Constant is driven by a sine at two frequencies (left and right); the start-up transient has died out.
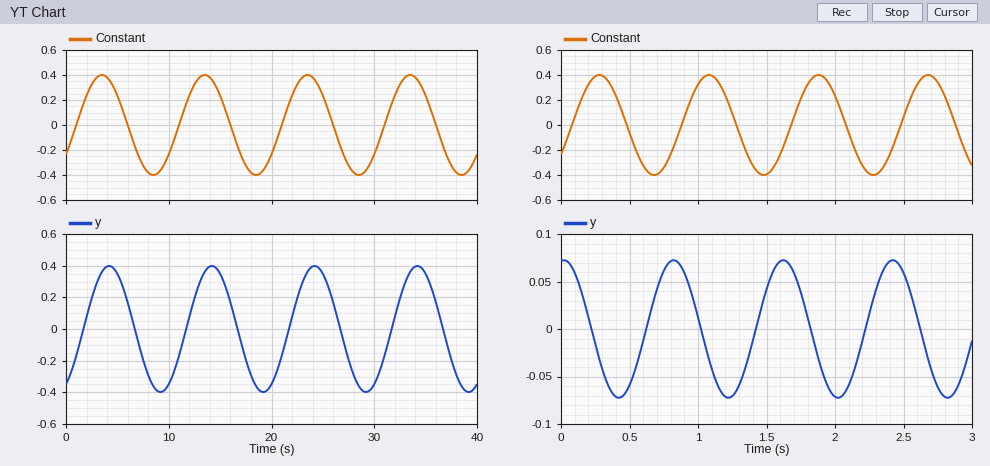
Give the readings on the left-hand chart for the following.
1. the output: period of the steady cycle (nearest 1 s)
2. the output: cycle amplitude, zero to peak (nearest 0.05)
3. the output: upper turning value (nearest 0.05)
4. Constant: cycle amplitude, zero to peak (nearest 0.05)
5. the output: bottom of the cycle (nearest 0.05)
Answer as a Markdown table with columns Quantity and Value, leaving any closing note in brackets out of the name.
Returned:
| Quantity | Value |
|---|---|
| the output: period of the steady cycle | 10 s |
| the output: cycle amplitude, zero to peak | 0.40 |
| the output: upper turning value | 0.40 |
| Constant: cycle amplitude, zero to peak | 0.40 |
| the output: bottom of the cycle | -0.40 |
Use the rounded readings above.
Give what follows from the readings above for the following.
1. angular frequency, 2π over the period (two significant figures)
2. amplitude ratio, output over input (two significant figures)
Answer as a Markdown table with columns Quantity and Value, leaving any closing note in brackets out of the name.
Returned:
| Quantity | Value |
|---|---|
| angular frequency, 2π over the period | 0.63 rad/s |
| amplitude ratio, output over input | 1.0 |
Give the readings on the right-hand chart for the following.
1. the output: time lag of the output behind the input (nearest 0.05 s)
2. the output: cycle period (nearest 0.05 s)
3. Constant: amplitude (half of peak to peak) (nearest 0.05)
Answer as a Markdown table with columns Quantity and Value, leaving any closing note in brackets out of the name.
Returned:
| Quantity | Value |
|---|---|
| the output: time lag of the output behind the input | 0.55 s |
| the output: cycle period | 0.80 s |
| Constant: amplitude (half of peak to peak) | 0.40 |
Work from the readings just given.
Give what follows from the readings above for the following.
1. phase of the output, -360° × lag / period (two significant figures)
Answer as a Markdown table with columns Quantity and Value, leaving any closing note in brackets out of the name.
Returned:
| Quantity | Value |
|---|---|
| phase of the output, -360° × lag / period | -250° |
